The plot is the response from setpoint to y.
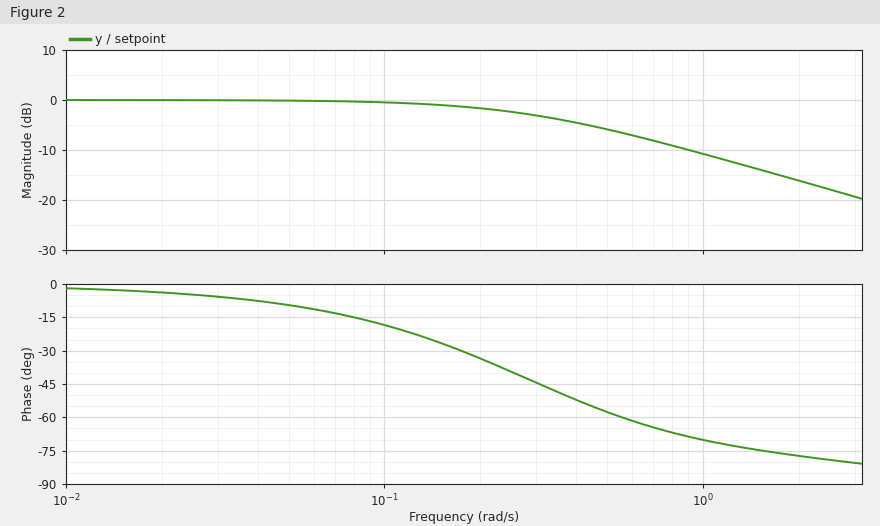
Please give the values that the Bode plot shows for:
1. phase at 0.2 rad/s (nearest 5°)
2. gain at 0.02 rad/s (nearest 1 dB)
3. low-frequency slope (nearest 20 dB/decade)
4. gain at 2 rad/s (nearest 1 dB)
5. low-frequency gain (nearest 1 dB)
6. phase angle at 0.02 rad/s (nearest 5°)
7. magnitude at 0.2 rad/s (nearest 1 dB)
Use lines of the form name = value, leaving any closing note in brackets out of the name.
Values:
phase at 0.2 rad/s = -35°
gain at 0.02 rad/s = 0 dB
low-frequency slope = 0 dB/decade
gain at 2 rad/s = -16 dB
low-frequency gain = 0 dB
phase angle at 0.02 rad/s = -5°
magnitude at 0.2 rad/s = -2 dB
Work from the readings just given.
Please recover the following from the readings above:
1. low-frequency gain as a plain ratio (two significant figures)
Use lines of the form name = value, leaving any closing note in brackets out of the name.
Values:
low-frequency gain as a plain ratio = 1.0
